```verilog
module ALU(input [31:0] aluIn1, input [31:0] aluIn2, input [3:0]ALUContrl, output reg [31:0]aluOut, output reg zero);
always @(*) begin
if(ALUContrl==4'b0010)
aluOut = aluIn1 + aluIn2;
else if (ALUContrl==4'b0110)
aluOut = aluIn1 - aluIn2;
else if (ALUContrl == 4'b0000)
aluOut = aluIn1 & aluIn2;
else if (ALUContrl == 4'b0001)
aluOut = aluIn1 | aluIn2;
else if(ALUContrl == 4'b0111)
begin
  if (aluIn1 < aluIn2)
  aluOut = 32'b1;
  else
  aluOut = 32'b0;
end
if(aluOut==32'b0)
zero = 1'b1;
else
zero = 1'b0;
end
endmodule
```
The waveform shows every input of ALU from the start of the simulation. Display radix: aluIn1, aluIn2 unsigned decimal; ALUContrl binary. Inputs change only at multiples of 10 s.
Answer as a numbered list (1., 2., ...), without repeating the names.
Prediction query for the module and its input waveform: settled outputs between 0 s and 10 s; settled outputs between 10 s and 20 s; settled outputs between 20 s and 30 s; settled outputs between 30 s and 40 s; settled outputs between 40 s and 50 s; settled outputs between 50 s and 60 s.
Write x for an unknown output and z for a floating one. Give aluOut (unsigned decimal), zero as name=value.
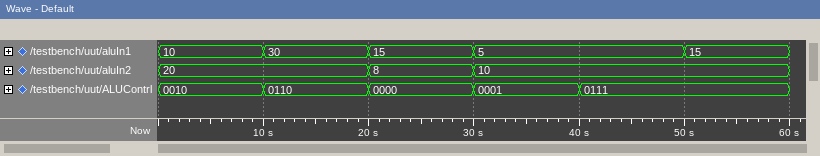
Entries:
1. aluOut=30, zero=0
2. aluOut=10, zero=0
3. aluOut=8, zero=0
4. aluOut=15, zero=0
5. aluOut=1, zero=0
6. aluOut=0, zero=1
